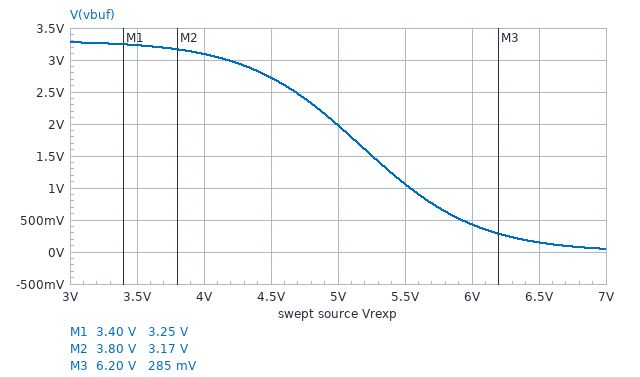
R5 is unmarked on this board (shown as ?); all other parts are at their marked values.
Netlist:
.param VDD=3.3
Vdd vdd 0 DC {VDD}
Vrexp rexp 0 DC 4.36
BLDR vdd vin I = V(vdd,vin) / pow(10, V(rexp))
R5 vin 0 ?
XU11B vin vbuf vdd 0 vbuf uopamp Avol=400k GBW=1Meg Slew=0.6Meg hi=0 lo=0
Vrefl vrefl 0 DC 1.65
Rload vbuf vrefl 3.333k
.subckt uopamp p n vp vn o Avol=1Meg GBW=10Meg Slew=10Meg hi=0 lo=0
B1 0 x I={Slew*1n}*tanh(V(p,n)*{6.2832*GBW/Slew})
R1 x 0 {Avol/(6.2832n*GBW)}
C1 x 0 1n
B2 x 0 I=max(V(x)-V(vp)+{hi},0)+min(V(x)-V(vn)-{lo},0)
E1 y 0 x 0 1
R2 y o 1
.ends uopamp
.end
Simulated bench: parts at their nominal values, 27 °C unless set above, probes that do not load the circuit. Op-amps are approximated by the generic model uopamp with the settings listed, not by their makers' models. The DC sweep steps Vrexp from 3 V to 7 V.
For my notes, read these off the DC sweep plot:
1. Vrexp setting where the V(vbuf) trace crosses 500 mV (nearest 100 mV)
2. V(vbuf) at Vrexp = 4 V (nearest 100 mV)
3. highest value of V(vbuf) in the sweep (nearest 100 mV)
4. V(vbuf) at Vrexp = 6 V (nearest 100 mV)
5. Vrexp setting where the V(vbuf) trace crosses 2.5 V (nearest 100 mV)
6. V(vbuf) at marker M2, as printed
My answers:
5.9 V
3.1 V
3.3 V
400 mV
4.7 V
3.17 V
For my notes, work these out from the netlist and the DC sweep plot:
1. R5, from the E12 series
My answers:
150 kΩ
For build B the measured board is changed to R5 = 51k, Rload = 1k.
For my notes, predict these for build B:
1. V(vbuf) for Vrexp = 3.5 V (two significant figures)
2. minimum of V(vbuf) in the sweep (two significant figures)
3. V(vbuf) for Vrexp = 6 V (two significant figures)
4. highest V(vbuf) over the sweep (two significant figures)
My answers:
3.1 V
17 mV
160 mV
3.2 V
